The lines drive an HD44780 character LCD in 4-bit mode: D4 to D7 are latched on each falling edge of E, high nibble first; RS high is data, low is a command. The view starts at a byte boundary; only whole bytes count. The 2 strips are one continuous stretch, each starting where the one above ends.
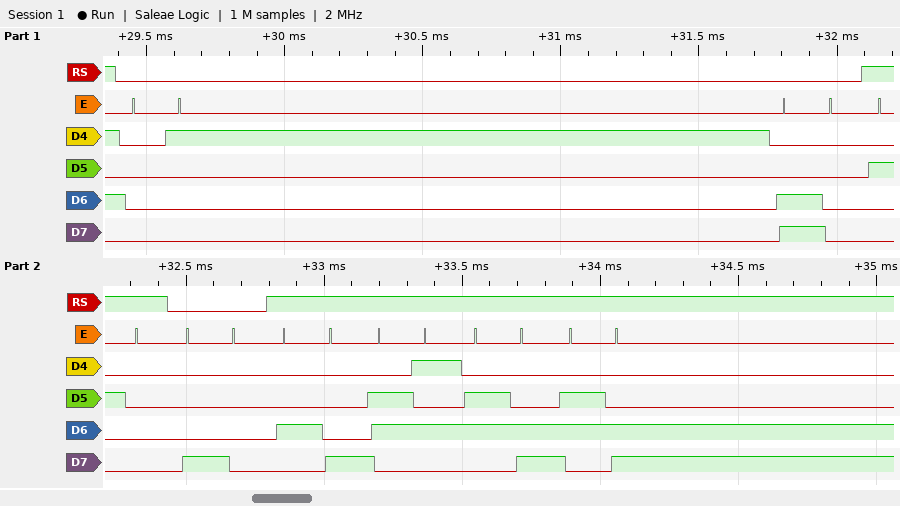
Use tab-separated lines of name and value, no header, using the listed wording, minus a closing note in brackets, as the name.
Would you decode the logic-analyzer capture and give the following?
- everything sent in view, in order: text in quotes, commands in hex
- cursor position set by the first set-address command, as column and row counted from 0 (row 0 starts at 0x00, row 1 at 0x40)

everything sent in view, in order: text in quotes, commands in hex	0x01 0xC0 " " 0x80 "Hell"
cursor position set by the first set-address command, as column and row counted from 0	column 0, row 1
